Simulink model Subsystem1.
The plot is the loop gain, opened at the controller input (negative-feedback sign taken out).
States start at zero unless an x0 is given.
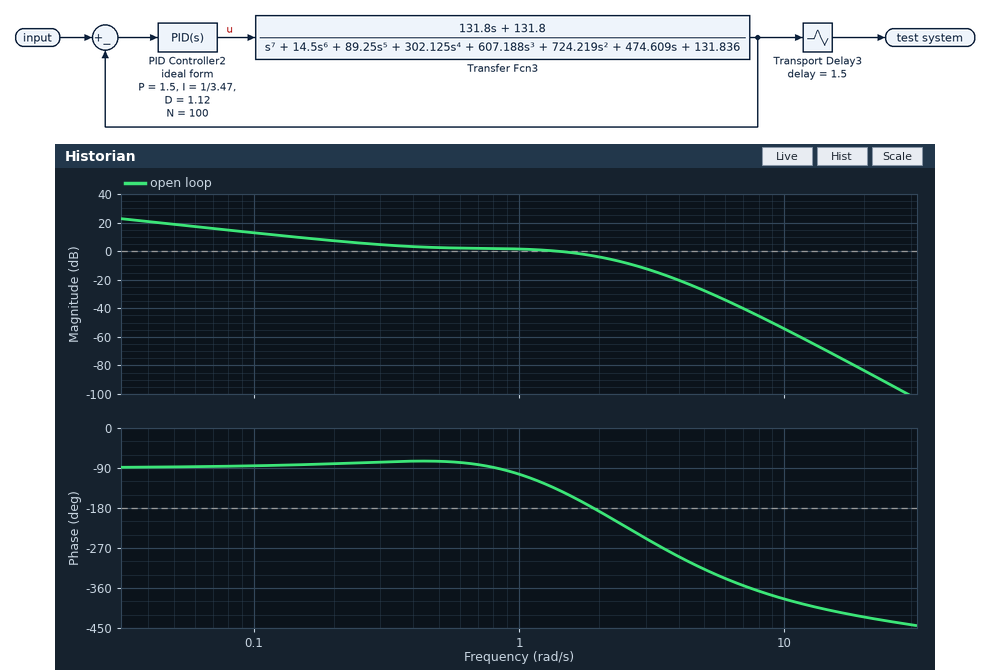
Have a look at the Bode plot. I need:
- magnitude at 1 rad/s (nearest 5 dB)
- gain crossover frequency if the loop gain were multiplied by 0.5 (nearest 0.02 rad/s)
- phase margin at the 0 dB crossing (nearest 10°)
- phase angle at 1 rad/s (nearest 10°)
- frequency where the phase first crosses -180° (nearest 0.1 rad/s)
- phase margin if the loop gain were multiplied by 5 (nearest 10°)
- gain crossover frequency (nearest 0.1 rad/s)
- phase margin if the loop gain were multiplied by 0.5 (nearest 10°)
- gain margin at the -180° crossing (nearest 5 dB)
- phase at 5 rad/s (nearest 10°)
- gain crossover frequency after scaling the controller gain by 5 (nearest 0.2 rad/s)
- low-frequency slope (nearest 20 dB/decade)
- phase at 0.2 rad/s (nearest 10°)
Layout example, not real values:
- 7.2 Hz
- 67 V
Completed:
- 0 dB
- 0.24 rad/s
- 40°
- -100°
- 1.9 rad/s
- -80°
- 1.4 rad/s
- 100°
- 5 dB
- -320°
- 3.2 rad/s
- -20 dB/decade
- -80°
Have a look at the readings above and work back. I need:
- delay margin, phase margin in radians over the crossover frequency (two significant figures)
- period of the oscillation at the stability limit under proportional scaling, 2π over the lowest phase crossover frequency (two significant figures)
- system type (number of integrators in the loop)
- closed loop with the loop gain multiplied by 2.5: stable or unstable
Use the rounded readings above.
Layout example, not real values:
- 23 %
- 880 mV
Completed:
- 0.50 s
- 3.3 s
- 1
- unstable
